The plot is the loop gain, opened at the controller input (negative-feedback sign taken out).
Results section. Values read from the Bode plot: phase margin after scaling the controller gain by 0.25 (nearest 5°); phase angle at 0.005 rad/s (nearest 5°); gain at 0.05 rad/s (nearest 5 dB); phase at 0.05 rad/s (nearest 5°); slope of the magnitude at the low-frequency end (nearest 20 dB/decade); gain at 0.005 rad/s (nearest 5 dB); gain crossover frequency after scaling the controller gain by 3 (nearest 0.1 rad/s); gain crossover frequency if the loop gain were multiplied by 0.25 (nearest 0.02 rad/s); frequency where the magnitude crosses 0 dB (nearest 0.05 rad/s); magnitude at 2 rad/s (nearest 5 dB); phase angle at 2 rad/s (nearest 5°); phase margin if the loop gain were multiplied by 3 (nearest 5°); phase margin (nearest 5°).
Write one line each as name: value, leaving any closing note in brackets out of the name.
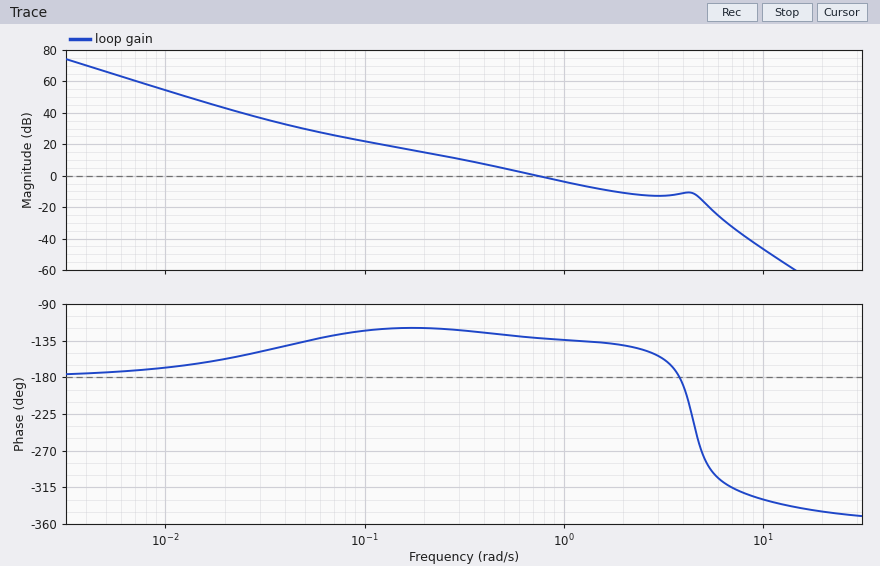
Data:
phase margin after scaling the controller gain by 0.25: 60°
phase angle at 0.005 rad/s: -175°
gain at 0.05 rad/s: 30 dB
phase at 0.05 rad/s: -135°
slope of the magnitude at the low-frequency end: -40 dB/decade
gain at 0.005 rad/s: 65 dB
gain crossover frequency after scaling the controller gain by 3: 1.7 rad/s
gain crossover frequency if the loop gain were multiplied by 0.25: 0.26 rad/s
frequency where the magnitude crosses 0 dB: 0.75 rad/s
magnitude at 2 rad/s: -10 dB
phase angle at 2 rad/s: -140°
phase margin if the loop gain were multiplied by 3: 40°
phase margin: 50°
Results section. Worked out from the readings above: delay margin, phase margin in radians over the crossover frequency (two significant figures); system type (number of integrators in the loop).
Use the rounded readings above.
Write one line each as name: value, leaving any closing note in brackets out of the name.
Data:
delay margin, phase margin in radians over the crossover frequency: 1.2 s
system type: 2
